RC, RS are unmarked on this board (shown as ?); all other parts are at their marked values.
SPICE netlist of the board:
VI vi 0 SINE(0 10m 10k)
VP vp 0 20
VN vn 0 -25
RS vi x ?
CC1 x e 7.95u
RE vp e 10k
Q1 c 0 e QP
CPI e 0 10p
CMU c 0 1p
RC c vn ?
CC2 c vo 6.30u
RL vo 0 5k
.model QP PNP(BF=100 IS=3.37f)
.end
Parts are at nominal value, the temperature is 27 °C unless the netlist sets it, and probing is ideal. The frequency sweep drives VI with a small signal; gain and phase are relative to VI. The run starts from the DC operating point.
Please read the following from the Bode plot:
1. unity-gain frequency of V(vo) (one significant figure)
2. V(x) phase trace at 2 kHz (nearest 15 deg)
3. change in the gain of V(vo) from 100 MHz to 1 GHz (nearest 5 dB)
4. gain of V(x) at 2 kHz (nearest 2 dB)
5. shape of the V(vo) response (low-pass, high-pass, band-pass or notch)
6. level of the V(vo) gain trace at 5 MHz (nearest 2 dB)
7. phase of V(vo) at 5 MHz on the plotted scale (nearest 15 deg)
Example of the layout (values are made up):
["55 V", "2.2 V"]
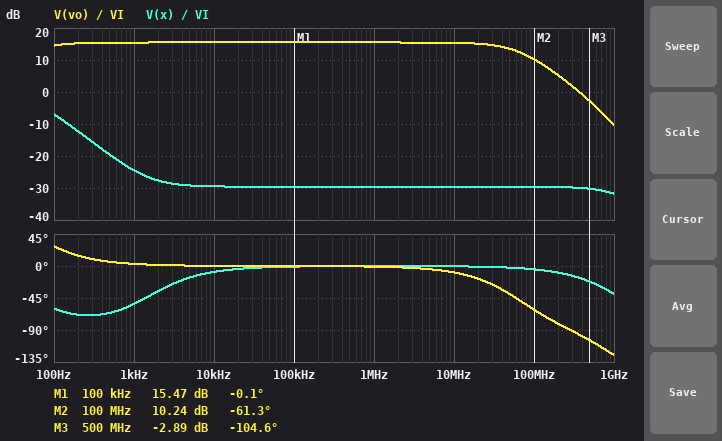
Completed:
["400 MHz", "-30 deg", "-20 dB", "-28 dB", "low-pass", "16 dB", "0 deg"]
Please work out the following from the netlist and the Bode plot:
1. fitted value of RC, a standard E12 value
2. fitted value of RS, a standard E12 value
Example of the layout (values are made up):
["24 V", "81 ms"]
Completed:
["4.7 kΩ", "390 Ω"]
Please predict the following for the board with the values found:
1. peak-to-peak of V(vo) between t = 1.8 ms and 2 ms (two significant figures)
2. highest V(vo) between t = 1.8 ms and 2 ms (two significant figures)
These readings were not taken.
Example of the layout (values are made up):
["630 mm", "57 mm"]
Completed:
["120 mV", "59 mV"]
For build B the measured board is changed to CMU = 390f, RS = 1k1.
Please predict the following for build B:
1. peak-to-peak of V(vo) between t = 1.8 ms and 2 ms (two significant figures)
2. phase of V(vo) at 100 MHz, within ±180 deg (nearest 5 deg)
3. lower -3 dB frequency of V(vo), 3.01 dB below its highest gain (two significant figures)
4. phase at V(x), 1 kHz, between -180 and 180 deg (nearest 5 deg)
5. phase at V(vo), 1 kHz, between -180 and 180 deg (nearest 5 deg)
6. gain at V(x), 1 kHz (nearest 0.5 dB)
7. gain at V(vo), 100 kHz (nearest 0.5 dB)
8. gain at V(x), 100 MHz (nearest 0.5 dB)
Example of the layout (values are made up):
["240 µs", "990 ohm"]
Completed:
["43 mV", "-35 deg", "18 Hz", "-55 deg", "0 deg", "-33.5 dB", "6.5 dB", "-38.5 dB"]
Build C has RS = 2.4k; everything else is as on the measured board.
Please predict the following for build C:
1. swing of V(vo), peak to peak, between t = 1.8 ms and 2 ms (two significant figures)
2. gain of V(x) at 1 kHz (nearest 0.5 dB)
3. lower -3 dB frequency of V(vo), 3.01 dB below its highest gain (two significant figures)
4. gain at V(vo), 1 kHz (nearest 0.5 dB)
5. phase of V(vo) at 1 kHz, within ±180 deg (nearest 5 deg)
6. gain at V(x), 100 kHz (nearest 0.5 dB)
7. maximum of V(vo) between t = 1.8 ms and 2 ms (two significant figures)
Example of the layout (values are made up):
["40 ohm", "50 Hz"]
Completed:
["20 mV", "-40.0 dB", "9.0 Hz", "0 dB", "0 deg", "-45.0 dB", "9.9 mV"]
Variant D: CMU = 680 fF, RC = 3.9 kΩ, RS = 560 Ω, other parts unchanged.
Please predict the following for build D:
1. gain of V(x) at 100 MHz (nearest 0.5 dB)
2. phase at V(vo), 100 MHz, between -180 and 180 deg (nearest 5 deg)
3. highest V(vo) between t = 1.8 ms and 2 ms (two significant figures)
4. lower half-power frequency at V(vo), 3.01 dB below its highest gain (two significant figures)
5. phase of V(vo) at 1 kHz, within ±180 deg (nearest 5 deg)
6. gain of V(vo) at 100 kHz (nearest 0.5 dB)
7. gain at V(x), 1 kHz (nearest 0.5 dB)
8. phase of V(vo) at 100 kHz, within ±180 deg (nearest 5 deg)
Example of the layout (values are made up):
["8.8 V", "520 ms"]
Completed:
["-32.5 dB", "-50 deg", "38 mV", "35 Hz", "0 deg", "11.5 dB", "-27.5 dB", "0 deg"]
